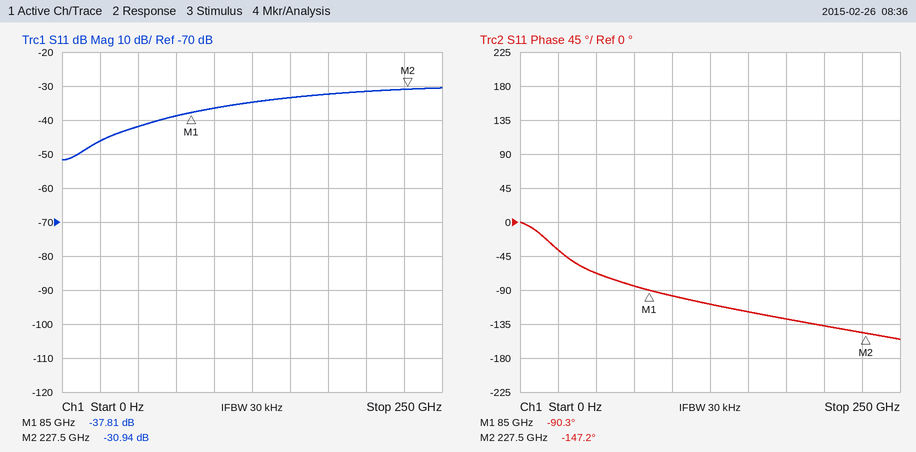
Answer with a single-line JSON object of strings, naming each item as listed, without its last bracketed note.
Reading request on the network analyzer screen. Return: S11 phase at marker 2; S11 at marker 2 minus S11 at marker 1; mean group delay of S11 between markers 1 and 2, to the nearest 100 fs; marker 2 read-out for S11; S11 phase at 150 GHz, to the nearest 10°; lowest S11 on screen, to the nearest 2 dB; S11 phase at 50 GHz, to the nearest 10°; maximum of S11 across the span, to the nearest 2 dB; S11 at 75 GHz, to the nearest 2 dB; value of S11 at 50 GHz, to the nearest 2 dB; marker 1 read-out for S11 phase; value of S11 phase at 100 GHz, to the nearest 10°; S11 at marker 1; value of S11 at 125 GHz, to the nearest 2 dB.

{"S11 phase at marker 2": "-147.2°", "S11 at marker 2 minus S11 at marker 1": "6.87 dB", "mean group delay of S11 between markers 1 and 2, to the nearest 100 fs": "1.1 ps", "marker 2 read-out for S11": "-30.94 dB", "S11 phase at 150 GHz, to the nearest 10°": "-120°", "lowest S11 on screen, to the nearest 2 dB": "-52 dB", "S11 phase at 50 GHz, to the nearest 10°": "-70°", "maximum of S11 across the span, to the nearest 2 dB": "-30 dB", "S11 at 75 GHz, to the nearest 2 dB": "-38 dB", "value of S11 at 50 GHz, to the nearest 2 dB": "-42 dB", "marker 1 read-out for S11 phase": "-90.3°", "value of S11 phase at 100 GHz, to the nearest 10°": "-100°", "S11 at marker 1": "-37.81 dB", "value of S11 at 125 GHz, to the nearest 2 dB": "-34 dB"}
